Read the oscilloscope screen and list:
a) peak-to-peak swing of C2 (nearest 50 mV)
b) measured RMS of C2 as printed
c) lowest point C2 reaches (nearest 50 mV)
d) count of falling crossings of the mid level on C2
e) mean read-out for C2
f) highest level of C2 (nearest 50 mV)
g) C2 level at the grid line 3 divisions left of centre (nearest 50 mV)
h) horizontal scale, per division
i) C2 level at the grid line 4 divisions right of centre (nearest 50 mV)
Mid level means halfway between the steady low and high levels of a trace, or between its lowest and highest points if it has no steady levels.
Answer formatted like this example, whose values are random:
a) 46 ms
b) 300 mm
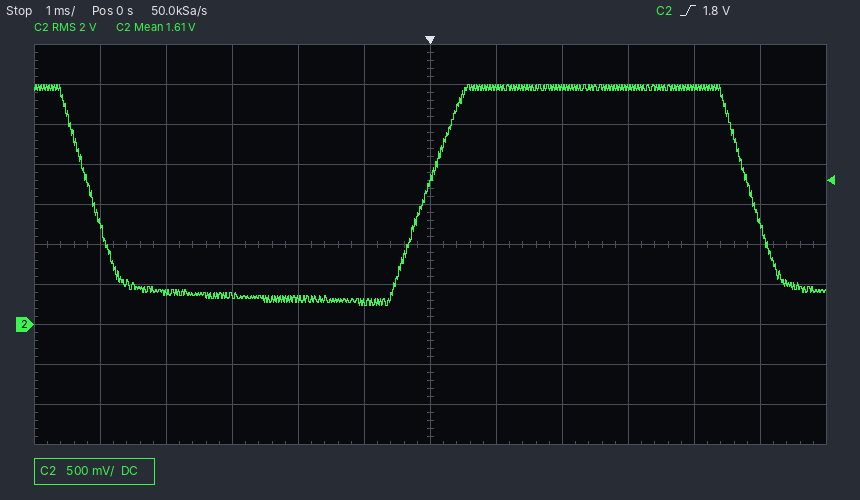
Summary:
a) 2.75 V
b) 2 V
c) 250 mV
d) 2
e) 1.61 V
f) 3.00 V
g) 350 mV
h) 1 ms
i) 2.95 V
